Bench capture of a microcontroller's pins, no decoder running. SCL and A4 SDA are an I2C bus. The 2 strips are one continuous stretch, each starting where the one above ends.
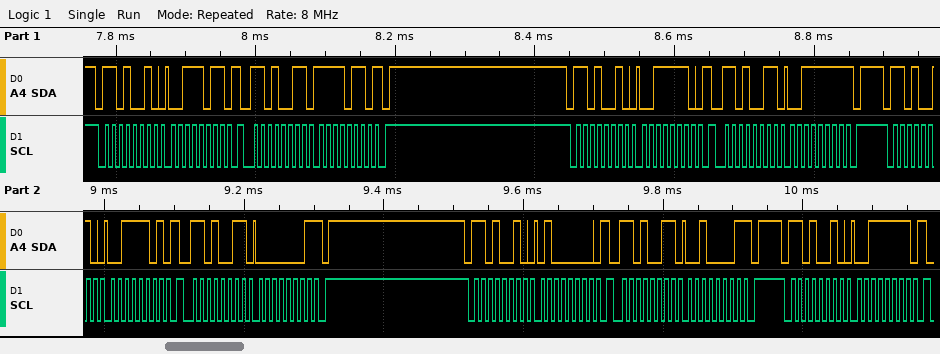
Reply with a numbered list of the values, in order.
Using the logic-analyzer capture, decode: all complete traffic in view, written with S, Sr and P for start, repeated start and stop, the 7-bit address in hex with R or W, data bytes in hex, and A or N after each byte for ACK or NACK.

1. S 69W A 3B A Sr 69R A F6 N P S 69W A 3E A Sr 69R A 3F N P S 69W A 3D A Sr 69R A 01 N P S 69W A 40 A Sr 69R A 21 N P S 69W A 3F A
